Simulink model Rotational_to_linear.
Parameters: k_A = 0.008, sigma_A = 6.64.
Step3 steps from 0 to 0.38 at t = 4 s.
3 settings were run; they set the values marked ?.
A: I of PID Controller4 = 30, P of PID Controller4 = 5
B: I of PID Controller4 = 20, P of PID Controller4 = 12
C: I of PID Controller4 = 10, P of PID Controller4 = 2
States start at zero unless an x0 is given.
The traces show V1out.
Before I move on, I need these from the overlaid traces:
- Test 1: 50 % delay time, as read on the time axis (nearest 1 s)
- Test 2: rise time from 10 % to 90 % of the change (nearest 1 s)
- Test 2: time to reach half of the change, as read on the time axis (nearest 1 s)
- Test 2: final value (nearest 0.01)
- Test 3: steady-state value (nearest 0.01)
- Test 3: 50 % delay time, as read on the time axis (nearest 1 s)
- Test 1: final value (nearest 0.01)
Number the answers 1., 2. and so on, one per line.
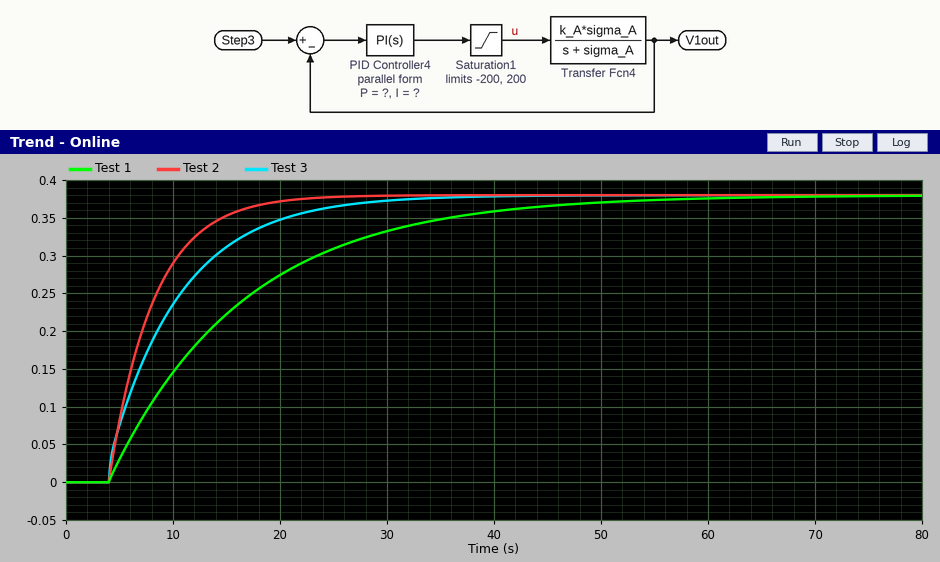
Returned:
1. 13 s
2. 9 s
3. 7 s
4. 0.38
5. 0.38
6. 8 s
7. 0.38
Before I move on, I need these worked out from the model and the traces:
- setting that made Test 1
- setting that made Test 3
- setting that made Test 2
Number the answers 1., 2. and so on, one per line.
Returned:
1. C
2. B
3. A
